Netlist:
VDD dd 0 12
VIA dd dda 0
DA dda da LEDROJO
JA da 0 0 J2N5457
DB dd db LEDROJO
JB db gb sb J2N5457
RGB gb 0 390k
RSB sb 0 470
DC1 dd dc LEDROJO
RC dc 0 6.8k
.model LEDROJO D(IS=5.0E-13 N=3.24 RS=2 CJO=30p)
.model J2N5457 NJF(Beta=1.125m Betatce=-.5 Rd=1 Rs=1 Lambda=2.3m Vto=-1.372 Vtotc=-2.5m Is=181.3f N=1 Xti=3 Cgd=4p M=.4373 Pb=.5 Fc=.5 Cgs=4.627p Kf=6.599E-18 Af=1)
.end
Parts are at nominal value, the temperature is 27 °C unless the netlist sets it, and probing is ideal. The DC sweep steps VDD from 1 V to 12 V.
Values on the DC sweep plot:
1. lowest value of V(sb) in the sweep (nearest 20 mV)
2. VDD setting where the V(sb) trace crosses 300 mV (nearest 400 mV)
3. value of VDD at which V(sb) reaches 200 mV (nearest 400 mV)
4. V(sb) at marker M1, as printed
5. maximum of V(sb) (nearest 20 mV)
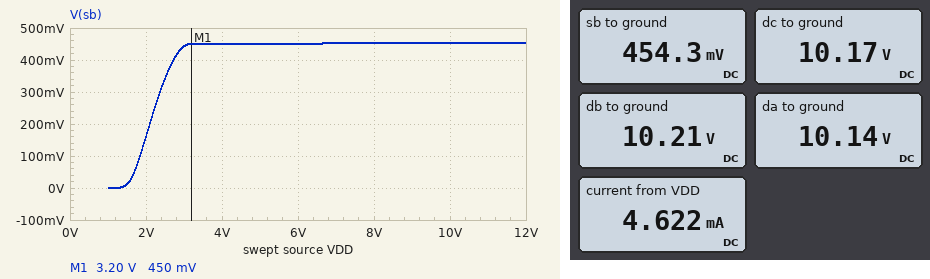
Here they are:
0 V
2.4 V
2.0 V
450 mV
460 mV
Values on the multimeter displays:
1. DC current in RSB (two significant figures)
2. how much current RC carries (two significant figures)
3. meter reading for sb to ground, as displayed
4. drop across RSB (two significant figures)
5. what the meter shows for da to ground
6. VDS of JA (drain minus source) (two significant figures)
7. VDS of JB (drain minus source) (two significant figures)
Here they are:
970 µA
1.5 mA
454.3 mV
450 mV
10.14 V
10 V
9.8 V
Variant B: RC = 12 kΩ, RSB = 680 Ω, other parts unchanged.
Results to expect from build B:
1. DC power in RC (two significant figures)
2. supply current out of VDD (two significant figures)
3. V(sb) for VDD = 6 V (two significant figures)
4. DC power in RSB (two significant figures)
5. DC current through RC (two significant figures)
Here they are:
8.7 mW
3.8 mA
540 mV
430 µW
850 µA
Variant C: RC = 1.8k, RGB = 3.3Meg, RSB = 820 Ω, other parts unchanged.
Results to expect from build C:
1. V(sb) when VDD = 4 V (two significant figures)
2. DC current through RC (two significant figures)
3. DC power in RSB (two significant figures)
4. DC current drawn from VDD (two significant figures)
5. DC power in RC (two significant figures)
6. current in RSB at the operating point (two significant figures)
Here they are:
580 mV
5.6 mA
420 µW
8.5 mA
56 mW
710 µA
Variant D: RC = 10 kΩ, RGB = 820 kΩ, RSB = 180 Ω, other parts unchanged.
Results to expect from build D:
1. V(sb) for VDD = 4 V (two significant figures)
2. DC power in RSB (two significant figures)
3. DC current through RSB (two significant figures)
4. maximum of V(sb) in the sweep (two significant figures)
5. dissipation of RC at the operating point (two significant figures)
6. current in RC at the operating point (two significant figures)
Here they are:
250 mV
370 µW
1.4 mA
260 mV
10 mW
1.0 mA
